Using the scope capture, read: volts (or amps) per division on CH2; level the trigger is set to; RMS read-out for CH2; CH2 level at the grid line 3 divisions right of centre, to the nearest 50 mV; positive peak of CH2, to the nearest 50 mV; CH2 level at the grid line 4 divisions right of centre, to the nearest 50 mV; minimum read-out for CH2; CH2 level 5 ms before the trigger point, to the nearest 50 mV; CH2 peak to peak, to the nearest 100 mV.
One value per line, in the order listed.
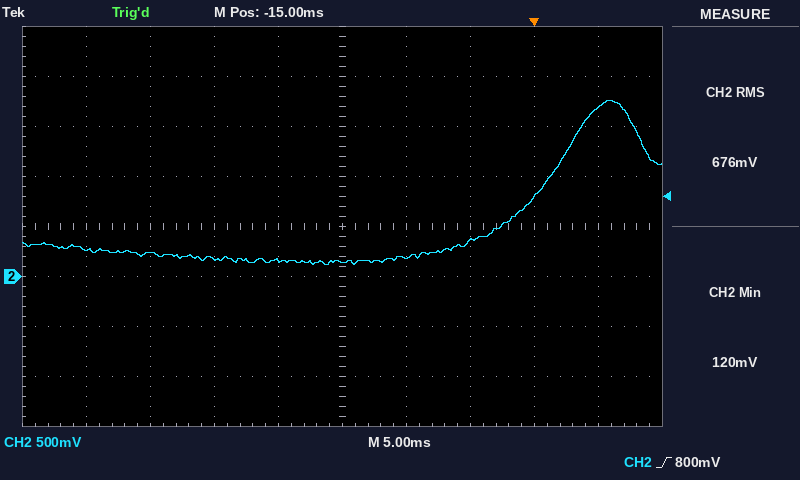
500 mV
800 mV
676 mV
800 mV
1.75 V
1.70 V
120 mV
350 mV
1.60 V
